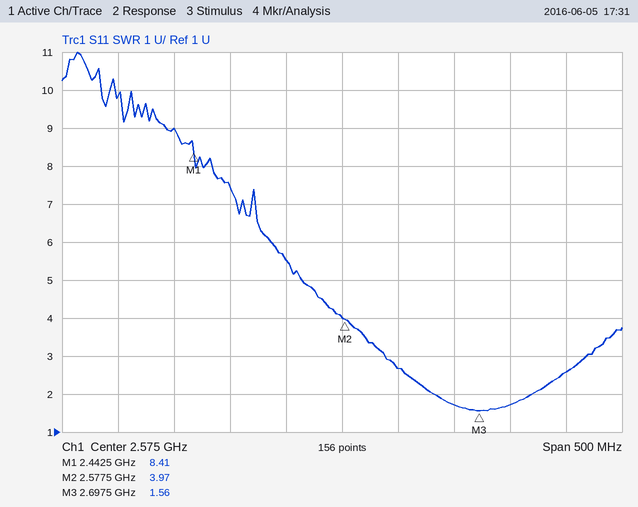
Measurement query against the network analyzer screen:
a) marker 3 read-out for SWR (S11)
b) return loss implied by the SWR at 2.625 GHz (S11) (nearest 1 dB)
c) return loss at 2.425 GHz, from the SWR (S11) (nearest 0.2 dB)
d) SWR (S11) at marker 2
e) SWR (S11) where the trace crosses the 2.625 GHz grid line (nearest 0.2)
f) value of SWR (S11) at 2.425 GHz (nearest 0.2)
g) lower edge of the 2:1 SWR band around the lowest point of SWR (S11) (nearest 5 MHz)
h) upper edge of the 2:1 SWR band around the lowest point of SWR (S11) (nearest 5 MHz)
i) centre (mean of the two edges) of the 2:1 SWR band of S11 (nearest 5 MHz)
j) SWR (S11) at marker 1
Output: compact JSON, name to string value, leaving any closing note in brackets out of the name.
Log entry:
{"marker 3 read-out for SWR": "1.56", "return loss implied by the SWR at 2.625 GHz (S11)": "7 dB", "return loss at 2.425 GHz, from the SWR (S11)": "2.0 dB", "SWR (S11) at marker 2": "3.97", "SWR (S11) where the trace crosses the 2.625 GHz grid line": "2.6", "value of SWR (S11) at 2.425 GHz": "9.0", "lower edge of the 2:1 SWR band around the lowest point of SWR (S11)": "2.655 GHz", "upper edge of the 2:1 SWR band around the lowest point of SWR (S11)": "2.745 GHz", "centre (mean of the two edges) of the 2:1 SWR band of S11": "2.700 GHz", "SWR (S11) at marker 1": "8.41"}
